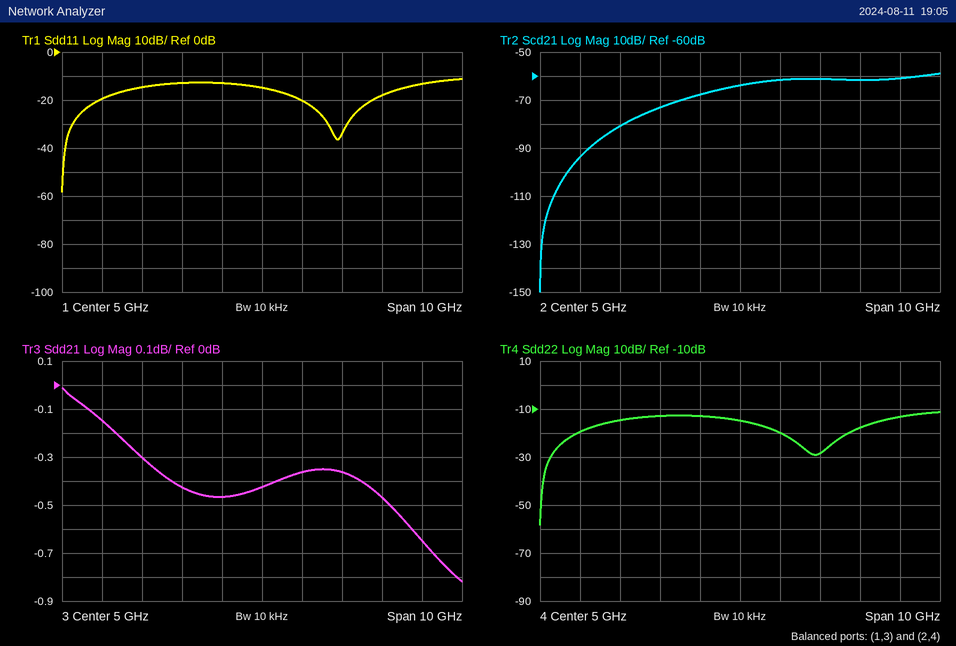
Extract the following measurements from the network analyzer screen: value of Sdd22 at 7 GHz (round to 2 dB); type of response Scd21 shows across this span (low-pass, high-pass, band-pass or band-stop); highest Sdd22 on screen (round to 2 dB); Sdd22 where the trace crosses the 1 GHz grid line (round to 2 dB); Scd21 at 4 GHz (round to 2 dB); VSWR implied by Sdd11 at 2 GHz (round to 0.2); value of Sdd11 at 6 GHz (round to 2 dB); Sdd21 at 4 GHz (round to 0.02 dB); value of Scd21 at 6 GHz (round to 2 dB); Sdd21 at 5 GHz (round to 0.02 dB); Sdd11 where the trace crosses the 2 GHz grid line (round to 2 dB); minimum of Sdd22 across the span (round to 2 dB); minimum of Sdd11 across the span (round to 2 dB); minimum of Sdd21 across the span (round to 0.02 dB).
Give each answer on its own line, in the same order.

-28 dB
high-pass
-12 dB
-20 dB
-68 dB
1.4
-20 dB
-0.46 dB
-62 dB
-0.42 dB
-14 dB
-58 dB
-58 dB
-0.82 dB
